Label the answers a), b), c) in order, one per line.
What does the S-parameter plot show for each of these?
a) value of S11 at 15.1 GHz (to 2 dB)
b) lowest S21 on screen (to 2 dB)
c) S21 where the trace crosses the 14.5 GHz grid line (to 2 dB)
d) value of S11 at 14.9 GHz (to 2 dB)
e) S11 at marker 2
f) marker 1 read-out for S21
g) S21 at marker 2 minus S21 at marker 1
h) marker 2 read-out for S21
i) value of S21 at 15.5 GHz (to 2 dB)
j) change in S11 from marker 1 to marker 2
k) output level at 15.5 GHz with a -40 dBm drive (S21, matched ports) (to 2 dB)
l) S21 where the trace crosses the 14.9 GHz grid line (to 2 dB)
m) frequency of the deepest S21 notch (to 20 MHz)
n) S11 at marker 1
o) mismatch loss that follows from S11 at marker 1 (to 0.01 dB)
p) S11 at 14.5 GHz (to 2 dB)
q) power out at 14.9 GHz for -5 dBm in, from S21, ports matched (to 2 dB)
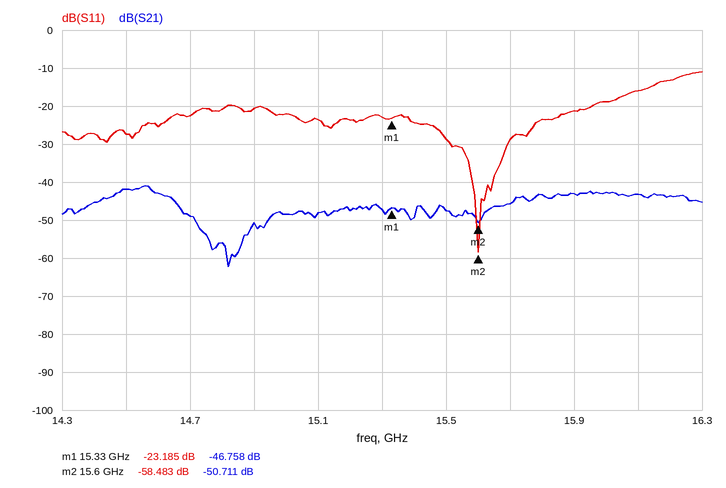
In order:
a) -24 dB
b) -62 dB
c) -42 dB
d) -20 dB
e) -58.483 dB
f) -46.758 dB
g) -3.953 dB
h) -50.711 dB
i) -48 dB
j) -35.298 dB
k) -88 dBm
l) -50 dB
m) 14.82 GHz
n) -23.185 dB
o) 0.02 dB
p) -28 dB
q) -56 dBm
